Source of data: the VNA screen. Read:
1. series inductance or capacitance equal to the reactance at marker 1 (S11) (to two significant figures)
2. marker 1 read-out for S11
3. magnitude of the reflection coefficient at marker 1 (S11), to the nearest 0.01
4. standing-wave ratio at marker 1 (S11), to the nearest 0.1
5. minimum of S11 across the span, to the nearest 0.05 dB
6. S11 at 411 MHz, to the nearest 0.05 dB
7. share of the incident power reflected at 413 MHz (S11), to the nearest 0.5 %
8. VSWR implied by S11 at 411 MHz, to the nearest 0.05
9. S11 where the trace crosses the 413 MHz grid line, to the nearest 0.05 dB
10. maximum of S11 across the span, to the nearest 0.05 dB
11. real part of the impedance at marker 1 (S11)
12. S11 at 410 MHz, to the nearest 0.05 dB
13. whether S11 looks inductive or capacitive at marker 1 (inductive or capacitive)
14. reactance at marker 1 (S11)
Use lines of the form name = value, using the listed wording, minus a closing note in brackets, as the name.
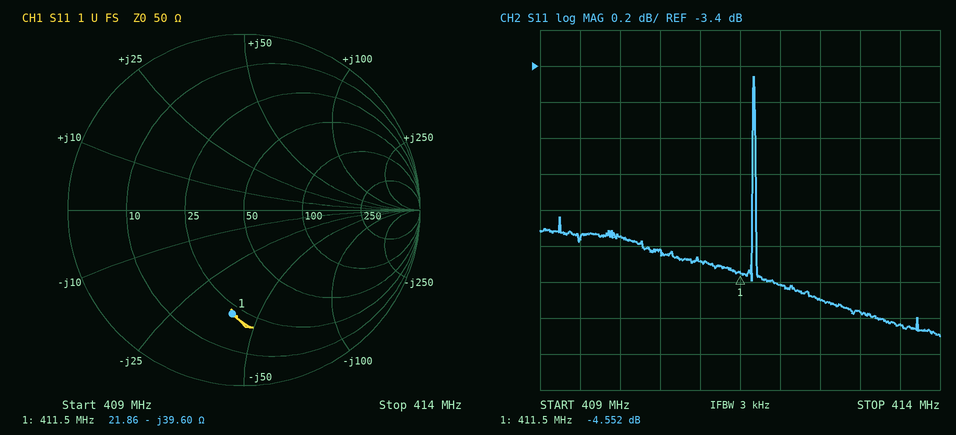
series inductance or capacitance equal to the reactance at marker 1 (S11) = 9.8 pF
marker 1 read-out for S11 = -4.552 dB
magnitude of the reflection coefficient at marker 1 (S11), to the nearest 0.01 = 0.59
standing-wave ratio at marker 1 (S11), to the nearest 0.1 = 3.9
minimum of S11 across the span, to the nearest 0.05 dB = -4.90 dB
S11 at 411 MHz, to the nearest 0.05 dB = -4.50 dB
share of the incident power reflected at 413 MHz (S11), to the nearest 0.5 % = 33.5 %
VSWR implied by S11 at 411 MHz, to the nearest 0.05 = 3.95
S11 where the trace crosses the 413 MHz grid line, to the nearest 0.05 dB = -4.75 dB
maximum of S11 across the span, to the nearest 0.05 dB = -3.45 dB
real part of the impedance at marker 1 = 21.86 Ω
S11 at 410 MHz, to the nearest 0.05 dB = -4.35 dB
whether S11 looks inductive or capacitive at marker 1 = capacitive
reactance at marker 1 = -39.60 Ω
